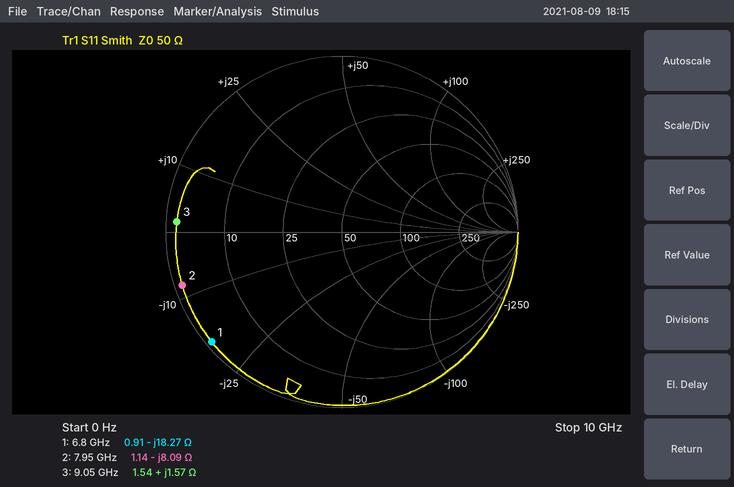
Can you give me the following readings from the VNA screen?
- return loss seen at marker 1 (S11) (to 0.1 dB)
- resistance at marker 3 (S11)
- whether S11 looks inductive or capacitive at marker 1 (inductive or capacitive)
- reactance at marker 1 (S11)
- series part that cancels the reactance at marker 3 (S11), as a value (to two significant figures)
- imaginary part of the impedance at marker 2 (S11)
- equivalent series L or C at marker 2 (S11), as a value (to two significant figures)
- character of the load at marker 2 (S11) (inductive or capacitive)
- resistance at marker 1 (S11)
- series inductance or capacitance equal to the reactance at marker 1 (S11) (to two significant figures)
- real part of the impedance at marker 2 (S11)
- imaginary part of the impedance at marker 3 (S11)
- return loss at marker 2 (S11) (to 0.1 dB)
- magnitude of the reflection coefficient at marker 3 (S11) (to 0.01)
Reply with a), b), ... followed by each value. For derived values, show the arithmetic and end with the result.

a) 0.3 dB
b) 1.54 Ω
c) capacitive
d) -18.27 Ω
e) C = 1/(2π × 9.05 GHz × 1.57 Ω) ≈ 11 pF
f) -8.09 Ω
g) C = 1/(2π × 7.95 GHz × 8.09 Ω) ≈ 2.5 pF
h) capacitive
i) 0.91 Ω
j) C = 1/(2π × 6.8 GHz × 18.27 Ω) ≈ 1.3 pF
k) 1.14 Ω
l) +1.57 Ω
m) 0.4 dB
n) 0.94
